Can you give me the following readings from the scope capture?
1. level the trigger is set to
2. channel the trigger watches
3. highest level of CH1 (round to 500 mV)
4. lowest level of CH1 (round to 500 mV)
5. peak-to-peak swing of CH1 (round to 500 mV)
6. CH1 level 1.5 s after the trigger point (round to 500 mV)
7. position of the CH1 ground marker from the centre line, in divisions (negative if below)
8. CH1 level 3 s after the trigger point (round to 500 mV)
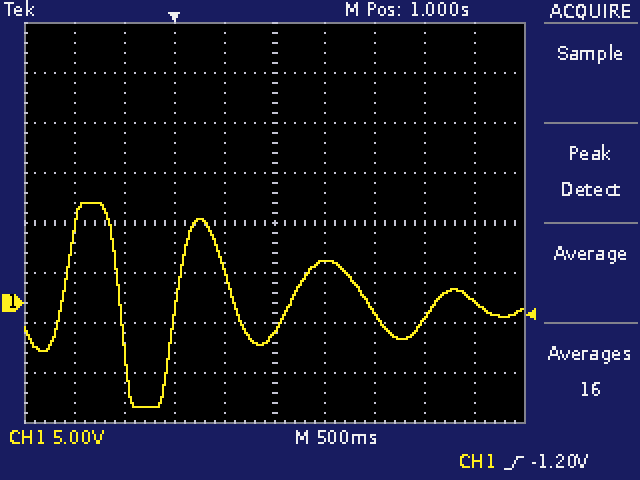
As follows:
-1.20 V
CH1
10.0 V
-10.5 V
20.5 V
4.0 V
-1.6 div
0.0 V
